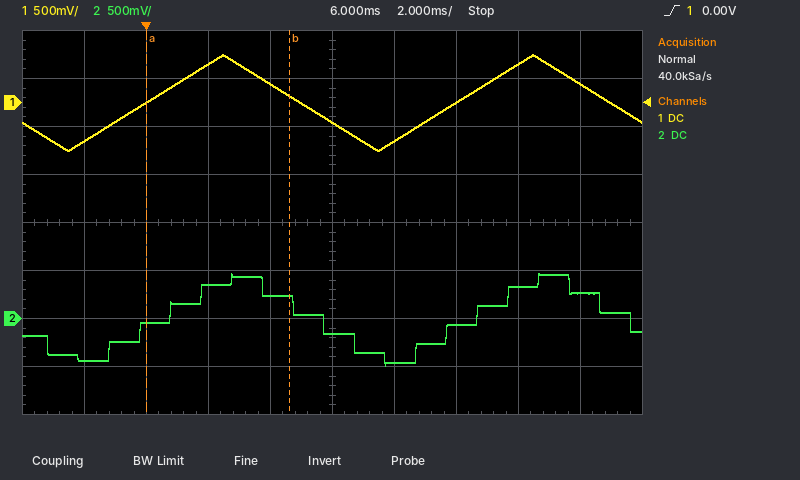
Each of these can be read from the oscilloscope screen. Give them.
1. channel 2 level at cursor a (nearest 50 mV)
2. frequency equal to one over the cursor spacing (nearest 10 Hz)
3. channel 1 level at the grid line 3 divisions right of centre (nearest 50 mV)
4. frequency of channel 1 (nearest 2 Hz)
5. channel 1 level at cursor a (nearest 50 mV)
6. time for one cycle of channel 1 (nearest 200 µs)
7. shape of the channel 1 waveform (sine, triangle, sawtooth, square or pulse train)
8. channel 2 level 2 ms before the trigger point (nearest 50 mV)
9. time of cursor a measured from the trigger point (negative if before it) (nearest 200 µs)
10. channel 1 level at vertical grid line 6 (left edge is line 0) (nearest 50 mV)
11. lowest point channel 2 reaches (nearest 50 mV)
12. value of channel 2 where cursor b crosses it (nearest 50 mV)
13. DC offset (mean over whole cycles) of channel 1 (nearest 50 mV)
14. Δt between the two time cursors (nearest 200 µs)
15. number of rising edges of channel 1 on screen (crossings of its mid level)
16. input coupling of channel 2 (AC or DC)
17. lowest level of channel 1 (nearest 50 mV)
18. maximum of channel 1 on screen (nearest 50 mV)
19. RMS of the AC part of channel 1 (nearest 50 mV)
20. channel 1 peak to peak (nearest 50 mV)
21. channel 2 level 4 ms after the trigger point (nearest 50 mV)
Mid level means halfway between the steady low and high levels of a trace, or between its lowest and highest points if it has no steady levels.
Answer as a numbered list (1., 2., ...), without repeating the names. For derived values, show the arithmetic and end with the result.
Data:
1. -50 mV
2. 1 / 4.6 ms ≈ 220 Hz
3. 400 mV
4. 1 / 10.0 ms ≈ 100 Hz
5. 0 mV
6. 10.0 ms
7. triangle
8. -450 mV
9. 0.0 ms
10. -400 mV
11. -500 mV
12. 200 mV
13. (500 mV + (-500 mV)) / 2 ≈ 0 mV
14. 4.6 ms
15. 2
16. DC
17. -500 mV
18. 500 mV
19. 1.00 V / (2√3) ≈ 289 mV, so 300 mV to the nearest 50 mV
20. 500 mV − (-500 mV) = 1.00 V
21. 250 mV
